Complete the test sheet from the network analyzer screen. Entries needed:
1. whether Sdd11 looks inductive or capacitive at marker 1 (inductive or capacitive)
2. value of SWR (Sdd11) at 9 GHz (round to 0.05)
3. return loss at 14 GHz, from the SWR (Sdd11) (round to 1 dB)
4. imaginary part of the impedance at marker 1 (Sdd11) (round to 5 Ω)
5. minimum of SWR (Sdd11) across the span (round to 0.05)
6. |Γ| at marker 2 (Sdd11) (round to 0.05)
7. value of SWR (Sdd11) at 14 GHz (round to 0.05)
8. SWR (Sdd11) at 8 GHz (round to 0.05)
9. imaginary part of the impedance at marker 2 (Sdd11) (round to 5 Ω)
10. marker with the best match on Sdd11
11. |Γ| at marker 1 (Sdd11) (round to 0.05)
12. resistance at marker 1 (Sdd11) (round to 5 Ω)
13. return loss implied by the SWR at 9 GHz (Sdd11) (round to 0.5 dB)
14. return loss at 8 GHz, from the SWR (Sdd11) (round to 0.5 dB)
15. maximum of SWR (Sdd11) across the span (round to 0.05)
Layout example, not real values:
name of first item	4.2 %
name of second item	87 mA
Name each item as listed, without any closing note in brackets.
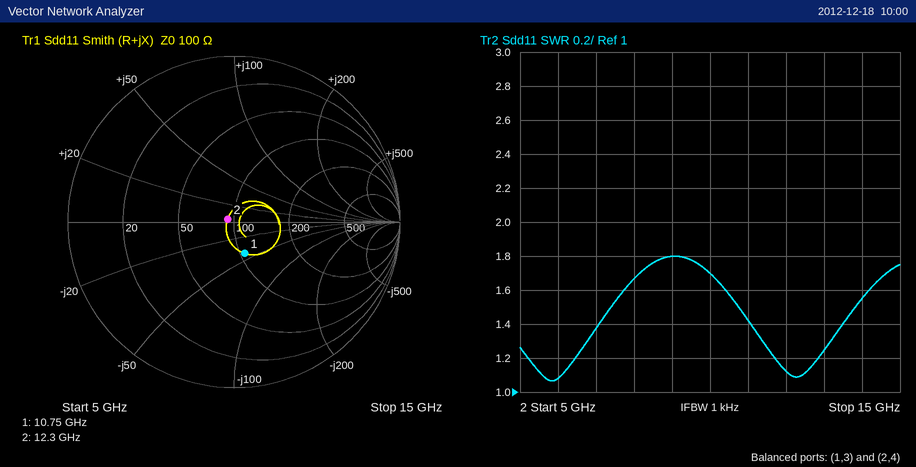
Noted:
whether Sdd11 looks inductive or capacitive at marker 1	capacitive
value of SWR (Sdd11) at 9 GHz	1.80
return loss at 14 GHz, from the SWR (Sdd11)	13 dB
imaginary part of the impedance at marker 1 (Sdd11)	-40 Ω
minimum of SWR (Sdd11) across the span	1.05
|Γ| at marker 2 (Sdd11)	0.05
value of SWR (Sdd11) at 14 GHz	1.55
SWR (Sdd11) at 8 GHz	1.65
imaginary part of the impedance at marker 2 (Sdd11)	+5 Ω
marker with the best match on Sdd11	marker 2
|Γ| at marker 1 (Sdd11)	0.20
resistance at marker 1 (Sdd11)	105 Ω
return loss implied by the SWR at 9 GHz (Sdd11)	11.0 dB
return loss at 8 GHz, from the SWR (Sdd11)	12.0 dB
maximum of SWR (Sdd11) across the span	1.80
